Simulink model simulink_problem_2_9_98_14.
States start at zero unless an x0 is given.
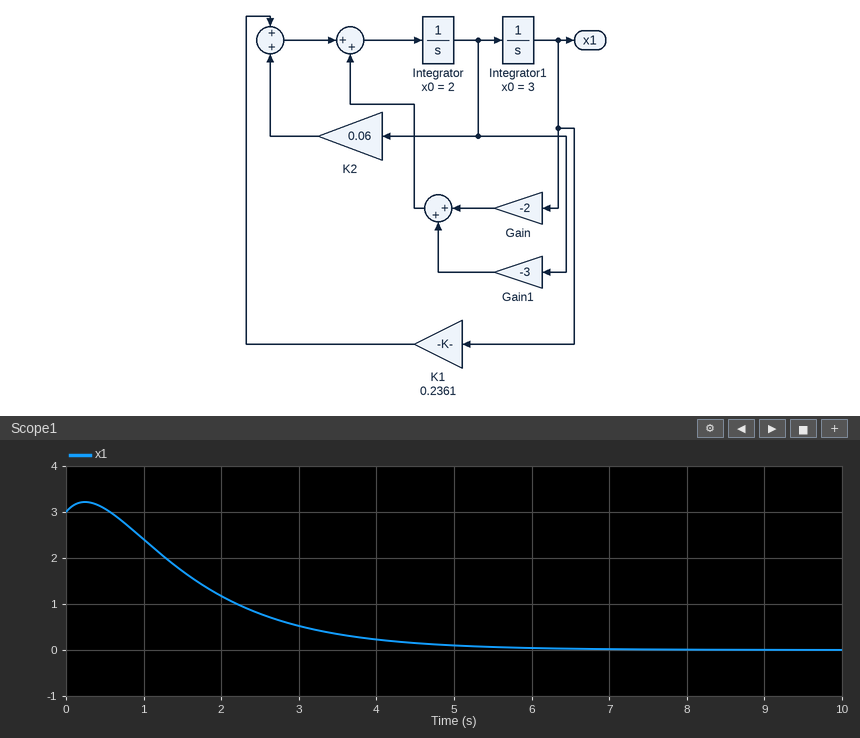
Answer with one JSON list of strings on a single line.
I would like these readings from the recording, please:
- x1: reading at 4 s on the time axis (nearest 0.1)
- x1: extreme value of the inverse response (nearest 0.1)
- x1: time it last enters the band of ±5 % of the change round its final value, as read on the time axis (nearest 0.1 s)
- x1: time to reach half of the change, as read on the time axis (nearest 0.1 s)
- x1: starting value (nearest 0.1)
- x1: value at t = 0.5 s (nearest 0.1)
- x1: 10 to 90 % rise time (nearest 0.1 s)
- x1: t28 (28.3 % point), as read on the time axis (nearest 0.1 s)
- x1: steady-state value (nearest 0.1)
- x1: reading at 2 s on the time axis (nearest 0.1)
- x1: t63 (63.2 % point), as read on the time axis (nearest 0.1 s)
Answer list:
["0.2", "3.2", "4.5 s", "1.7 s", "3.0", "3.1", "2.9 s", "1.2 s", "0.0", "1.2", "2.1 s"]
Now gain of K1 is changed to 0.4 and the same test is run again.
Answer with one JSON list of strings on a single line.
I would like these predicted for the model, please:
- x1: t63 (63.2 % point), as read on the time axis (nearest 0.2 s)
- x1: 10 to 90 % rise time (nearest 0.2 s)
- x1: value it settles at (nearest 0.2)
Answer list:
["2.2 s", "3.2 s", "0.0"]
